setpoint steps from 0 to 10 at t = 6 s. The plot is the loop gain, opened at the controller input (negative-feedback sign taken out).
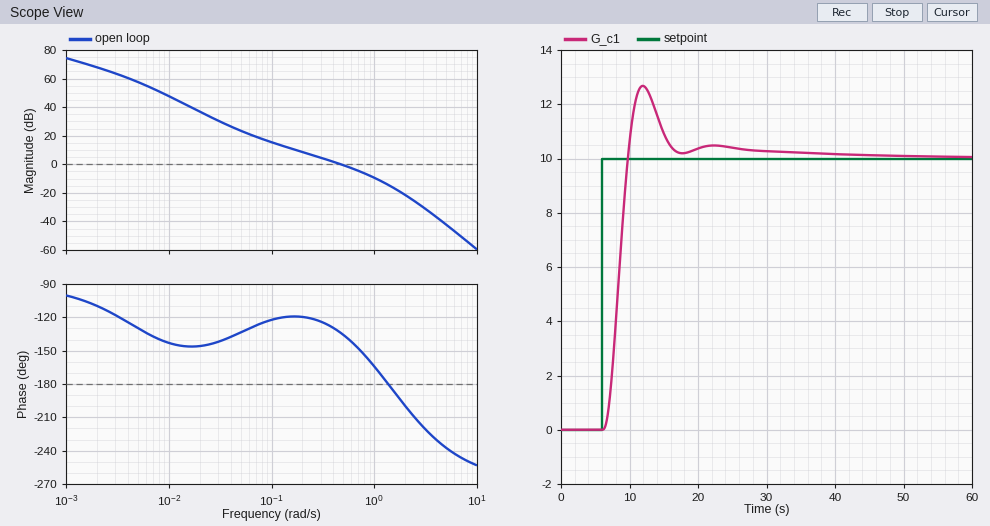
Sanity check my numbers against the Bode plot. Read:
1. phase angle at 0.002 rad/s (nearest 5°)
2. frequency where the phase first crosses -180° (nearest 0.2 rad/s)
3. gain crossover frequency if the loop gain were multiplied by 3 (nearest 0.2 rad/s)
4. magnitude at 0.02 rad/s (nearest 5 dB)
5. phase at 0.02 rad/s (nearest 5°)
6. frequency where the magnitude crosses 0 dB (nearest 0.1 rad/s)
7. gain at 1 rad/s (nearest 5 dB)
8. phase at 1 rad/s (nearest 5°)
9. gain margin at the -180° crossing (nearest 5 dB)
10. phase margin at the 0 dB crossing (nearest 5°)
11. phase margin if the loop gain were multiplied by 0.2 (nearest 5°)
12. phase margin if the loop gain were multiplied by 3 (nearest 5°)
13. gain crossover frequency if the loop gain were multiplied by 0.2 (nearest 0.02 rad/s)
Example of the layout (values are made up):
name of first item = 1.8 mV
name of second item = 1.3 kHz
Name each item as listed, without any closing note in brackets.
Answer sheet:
phase angle at 0.002 rad/s = -110°
frequency where the phase first crosses -180° = 1.4 rad/s
gain crossover frequency if the loop gain were multiplied by 3 = 1.0 rad/s
magnitude at 0.02 rad/s = 35 dB
phase at 0.02 rad/s = -145°
frequency where the magnitude crosses 0 dB = 0.5 rad/s
gain at 1 rad/s = -10 dB
phase at 1 rad/s = -165°
gain margin at the -180° crossing = 15 dB
phase margin at the 0 dB crossing = 45°
phase margin if the loop gain were multiplied by 0.2 = 60°
phase margin if the loop gain were multiplied by 3 = 15°
gain crossover frequency if the loop gain were multiplied by 0.2 = 0.12 rad/s
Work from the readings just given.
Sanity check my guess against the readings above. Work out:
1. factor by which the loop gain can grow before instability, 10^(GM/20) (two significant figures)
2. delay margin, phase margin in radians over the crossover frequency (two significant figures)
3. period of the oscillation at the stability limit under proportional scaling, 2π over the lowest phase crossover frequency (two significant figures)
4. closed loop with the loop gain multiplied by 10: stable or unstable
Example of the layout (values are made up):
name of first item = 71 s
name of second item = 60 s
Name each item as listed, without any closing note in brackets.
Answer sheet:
factor by which the loop gain can grow before instability, 10^(GM/20) = 5.6
delay margin, phase margin in radians over the crossover frequency = 1.6 s
period of the oscillation at the stability limit under proportional scaling, 2π over the lowest phase crossover frequency = 4.5 s
closed loop with the loop gain multiplied by 10: stable or unstable = unstable
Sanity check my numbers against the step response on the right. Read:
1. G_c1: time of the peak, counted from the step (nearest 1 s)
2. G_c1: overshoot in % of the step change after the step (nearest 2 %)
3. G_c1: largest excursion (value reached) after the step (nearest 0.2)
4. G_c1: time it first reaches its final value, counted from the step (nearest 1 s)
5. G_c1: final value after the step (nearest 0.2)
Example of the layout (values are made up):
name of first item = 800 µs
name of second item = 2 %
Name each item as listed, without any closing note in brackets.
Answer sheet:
G_c1: time of the peak, counted from the step = 6 s
G_c1: overshoot in % of the step change after the step = 26 %
G_c1: largest excursion (value reached) after the step = 12.6
G_c1: time it first reaches its final value, counted from the step = 4 s
G_c1: final value after the step = 10.0
